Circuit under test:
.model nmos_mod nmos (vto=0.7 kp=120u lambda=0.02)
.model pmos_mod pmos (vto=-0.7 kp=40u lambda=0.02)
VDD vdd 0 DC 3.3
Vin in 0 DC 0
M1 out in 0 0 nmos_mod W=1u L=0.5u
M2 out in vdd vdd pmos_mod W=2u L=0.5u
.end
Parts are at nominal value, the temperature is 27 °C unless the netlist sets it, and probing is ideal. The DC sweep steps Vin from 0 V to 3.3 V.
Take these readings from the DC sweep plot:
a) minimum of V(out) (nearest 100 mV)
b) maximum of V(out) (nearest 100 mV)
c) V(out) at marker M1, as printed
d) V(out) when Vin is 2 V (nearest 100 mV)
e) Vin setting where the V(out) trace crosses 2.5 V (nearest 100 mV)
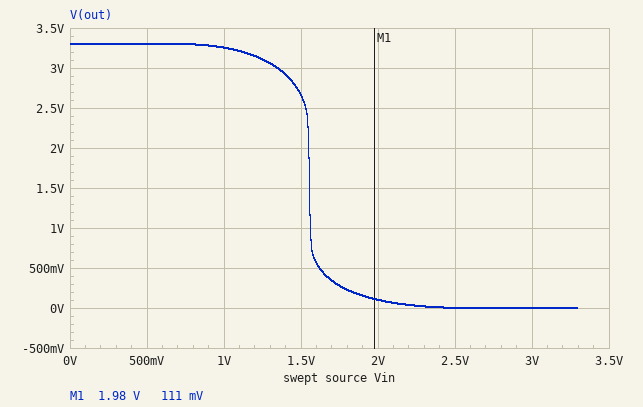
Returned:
0 V
3.3 V
111 mV
100 mV
1.5 V
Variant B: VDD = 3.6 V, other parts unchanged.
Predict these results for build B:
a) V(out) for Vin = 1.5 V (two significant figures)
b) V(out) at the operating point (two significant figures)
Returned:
3.2 V
3.6 V
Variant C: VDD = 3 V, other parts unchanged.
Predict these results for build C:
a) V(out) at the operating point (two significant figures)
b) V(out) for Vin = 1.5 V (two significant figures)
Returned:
3.0 V
360 mV
